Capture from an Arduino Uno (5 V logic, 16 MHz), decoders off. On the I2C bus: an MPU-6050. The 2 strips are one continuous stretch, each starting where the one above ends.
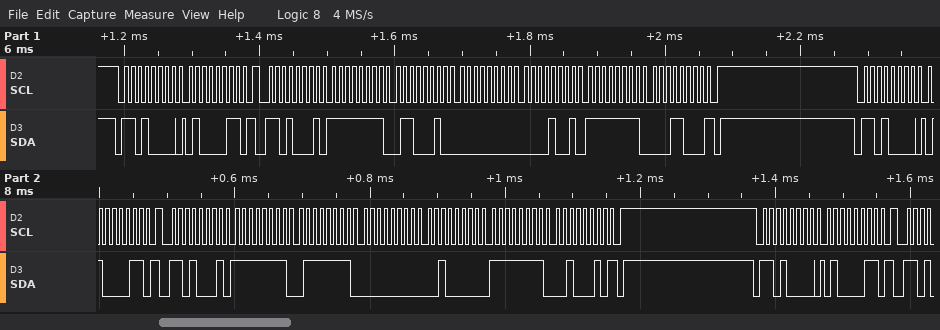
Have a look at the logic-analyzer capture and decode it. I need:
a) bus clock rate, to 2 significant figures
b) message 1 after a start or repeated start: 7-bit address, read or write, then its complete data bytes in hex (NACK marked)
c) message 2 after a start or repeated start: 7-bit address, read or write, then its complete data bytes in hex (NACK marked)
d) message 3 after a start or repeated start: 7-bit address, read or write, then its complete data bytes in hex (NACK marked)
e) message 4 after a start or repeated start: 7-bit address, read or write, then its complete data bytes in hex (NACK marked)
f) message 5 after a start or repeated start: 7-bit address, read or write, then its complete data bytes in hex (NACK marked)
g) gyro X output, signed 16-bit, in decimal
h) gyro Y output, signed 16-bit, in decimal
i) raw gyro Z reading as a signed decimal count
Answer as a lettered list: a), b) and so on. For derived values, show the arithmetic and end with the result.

a) 100 kHz
b) 0x68 write: 43
c) 0x68 read: FF 62 00 09 FF 18 NACK
d) 0x68 write: 43
e) 0x68 read: FF 7F 00 20 FF 22 NACK
f) 0x68 write: 43
g) 0xFF62 = -158
h) 0x0009 = 9
i) 0xFF18 = -232
